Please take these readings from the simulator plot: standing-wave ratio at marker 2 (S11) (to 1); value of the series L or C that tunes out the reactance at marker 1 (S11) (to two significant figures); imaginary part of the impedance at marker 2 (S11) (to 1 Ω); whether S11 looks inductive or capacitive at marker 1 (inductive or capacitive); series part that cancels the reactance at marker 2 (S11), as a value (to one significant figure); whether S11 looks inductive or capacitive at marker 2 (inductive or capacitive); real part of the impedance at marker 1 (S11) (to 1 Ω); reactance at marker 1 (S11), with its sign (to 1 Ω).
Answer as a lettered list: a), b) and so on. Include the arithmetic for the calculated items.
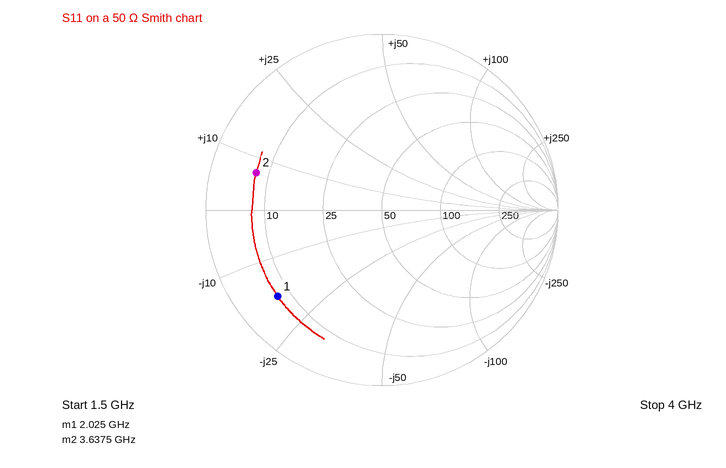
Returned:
a) 7
b) L = 18 Ω/(2π × 2.025 GHz) ≈ 1.4 nH
c) +7 Ω
d) capacitive
e) C = 1/(2π × 3.6375 GHz × 7 Ω) ≈ 6 pF
f) inductive
g) 7 Ω
h) -18 Ω
